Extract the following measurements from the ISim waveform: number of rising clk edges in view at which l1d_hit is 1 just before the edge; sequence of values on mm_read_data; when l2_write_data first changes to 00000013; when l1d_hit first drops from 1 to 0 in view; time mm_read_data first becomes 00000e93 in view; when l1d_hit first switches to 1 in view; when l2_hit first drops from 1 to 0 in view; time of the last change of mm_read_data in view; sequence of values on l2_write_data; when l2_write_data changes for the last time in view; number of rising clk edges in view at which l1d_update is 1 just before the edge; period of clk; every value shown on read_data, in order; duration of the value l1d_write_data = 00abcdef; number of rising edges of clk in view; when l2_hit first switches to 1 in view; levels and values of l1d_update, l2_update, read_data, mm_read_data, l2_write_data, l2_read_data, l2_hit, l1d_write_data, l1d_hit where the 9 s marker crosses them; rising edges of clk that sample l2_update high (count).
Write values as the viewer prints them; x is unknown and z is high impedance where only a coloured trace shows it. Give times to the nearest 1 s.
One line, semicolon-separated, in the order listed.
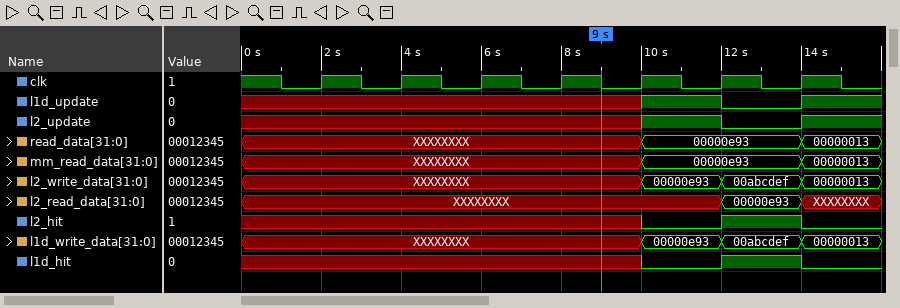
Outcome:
1; XXXXXXXX, 00000e93, 00000013; 14 s; 14 s; 10 s; 12 s; 14 s; 14 s; XXXXXXXX, 00000e93, 00abcdef, 00000013; 14 s; 1; 2 s; XXXXXXXX, 00000e93, 00000013; 2 s; 7; 12 s; l1d_update=x, l2_update=x, read_data=XXXXXXXX, mm_read_data=XXXXXXXX, l2_write_data=XXXXXXXX, l2_read_data=XXXXXXXX, l2_hit=x, l1d_write_data=XXXXXXXX, l1d_hit=x; 1
